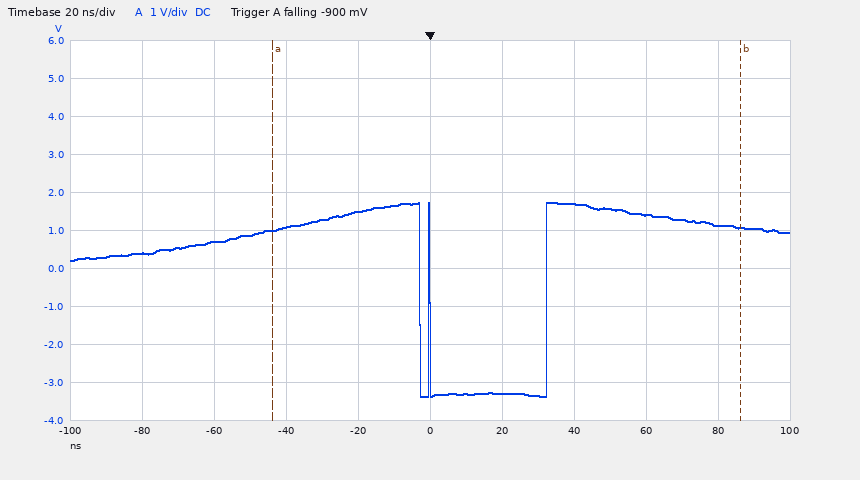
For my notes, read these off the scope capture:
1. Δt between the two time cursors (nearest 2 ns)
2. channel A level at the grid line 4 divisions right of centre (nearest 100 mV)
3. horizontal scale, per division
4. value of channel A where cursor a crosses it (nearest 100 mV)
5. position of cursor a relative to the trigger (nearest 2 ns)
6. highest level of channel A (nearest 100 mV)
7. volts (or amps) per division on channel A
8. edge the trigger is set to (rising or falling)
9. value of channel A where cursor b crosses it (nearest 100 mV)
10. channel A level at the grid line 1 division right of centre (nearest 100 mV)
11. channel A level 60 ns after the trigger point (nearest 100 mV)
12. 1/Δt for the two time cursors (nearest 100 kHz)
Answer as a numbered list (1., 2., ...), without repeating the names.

1. 130 ns
2. 1.1 V
3. 20 ns
4. 1.0 V
5. -44 ns
6. 1.7 V
7. 1 V
8. falling
9. 1.1 V
10. -3.3 V
11. 1.4 V
12. 7.7 MHz
